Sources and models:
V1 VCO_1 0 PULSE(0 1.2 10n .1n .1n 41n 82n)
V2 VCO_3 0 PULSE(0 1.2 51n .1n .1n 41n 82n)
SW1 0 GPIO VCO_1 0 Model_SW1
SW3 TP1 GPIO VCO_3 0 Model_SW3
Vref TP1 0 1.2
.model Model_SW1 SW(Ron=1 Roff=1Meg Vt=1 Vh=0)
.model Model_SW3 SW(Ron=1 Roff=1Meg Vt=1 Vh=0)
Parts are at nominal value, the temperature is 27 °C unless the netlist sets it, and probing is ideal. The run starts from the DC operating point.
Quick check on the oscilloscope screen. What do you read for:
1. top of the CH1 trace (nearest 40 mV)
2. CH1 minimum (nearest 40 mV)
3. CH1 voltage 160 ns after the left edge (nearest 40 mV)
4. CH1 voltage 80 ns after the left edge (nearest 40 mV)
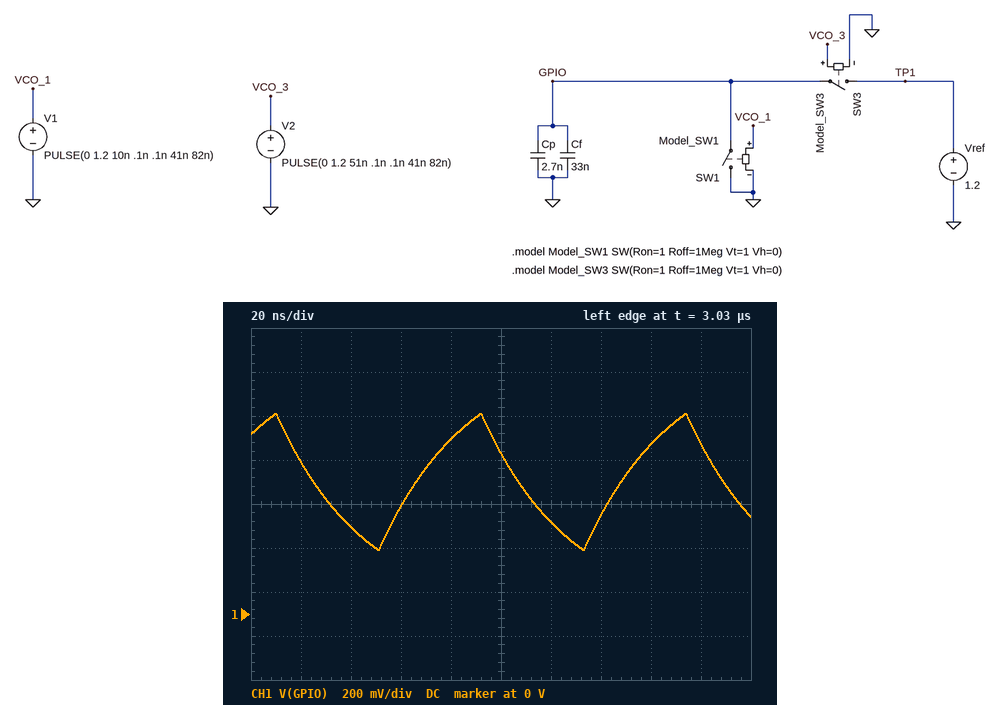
920 mV
280 mV
760 mV
800 mV
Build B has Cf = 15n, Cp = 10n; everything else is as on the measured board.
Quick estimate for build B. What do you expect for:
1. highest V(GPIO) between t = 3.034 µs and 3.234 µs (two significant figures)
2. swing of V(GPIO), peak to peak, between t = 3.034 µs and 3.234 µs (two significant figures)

1.0 V
810 mV
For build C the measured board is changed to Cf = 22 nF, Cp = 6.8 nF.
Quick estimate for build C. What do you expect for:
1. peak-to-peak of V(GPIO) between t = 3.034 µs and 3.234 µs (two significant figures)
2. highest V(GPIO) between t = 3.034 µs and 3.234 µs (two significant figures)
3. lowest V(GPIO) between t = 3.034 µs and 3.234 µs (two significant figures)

730 mV
970 mV
230 mV
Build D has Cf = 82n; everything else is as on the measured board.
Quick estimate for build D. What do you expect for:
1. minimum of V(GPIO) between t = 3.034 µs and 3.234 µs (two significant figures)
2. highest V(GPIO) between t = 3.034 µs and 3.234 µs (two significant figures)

460 mV
740 mV
